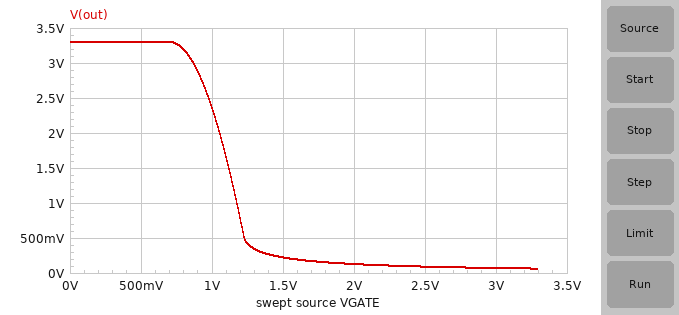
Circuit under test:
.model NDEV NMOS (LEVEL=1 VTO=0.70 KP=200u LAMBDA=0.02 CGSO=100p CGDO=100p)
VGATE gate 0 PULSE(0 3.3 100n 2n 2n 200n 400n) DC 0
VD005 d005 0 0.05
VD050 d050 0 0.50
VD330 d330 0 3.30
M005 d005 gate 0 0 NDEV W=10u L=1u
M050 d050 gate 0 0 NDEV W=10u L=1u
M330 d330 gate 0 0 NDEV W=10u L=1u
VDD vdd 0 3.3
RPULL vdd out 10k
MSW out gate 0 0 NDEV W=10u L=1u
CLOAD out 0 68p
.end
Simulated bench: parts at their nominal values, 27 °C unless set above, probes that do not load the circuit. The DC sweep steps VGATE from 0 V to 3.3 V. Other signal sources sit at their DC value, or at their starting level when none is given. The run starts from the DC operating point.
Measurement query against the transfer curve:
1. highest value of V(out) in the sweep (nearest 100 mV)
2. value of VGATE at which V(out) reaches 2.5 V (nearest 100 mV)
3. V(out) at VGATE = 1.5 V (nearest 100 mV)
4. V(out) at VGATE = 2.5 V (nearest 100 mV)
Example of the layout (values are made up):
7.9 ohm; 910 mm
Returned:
3.3 V; 1.0 V; 200 mV; 100 mV
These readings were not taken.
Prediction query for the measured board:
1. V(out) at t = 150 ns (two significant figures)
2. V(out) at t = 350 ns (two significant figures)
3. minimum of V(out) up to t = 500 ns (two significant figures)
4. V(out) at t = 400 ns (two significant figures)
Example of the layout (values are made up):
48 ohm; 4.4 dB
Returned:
250 mV; 280 mV; 63 mV; 490 mV
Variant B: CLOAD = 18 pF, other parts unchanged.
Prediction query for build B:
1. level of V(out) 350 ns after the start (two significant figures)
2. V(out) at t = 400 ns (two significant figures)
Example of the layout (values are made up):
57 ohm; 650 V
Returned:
810 mV; 1.4 V
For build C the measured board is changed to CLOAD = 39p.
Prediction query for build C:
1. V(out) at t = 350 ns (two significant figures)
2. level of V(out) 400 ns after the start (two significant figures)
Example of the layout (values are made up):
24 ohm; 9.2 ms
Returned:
430 mV; 780 mV
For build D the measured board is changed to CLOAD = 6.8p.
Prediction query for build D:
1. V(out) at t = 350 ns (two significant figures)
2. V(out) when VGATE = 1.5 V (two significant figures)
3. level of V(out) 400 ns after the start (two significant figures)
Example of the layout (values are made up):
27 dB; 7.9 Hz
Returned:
1.7 V; 220 mV; 2.5 V
